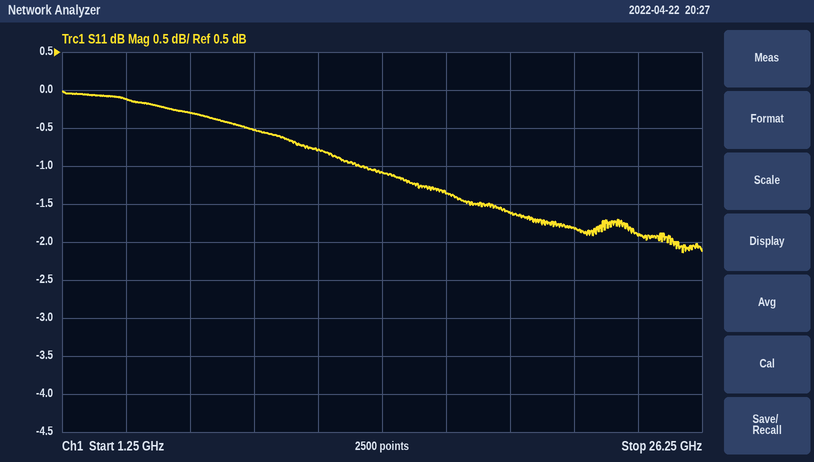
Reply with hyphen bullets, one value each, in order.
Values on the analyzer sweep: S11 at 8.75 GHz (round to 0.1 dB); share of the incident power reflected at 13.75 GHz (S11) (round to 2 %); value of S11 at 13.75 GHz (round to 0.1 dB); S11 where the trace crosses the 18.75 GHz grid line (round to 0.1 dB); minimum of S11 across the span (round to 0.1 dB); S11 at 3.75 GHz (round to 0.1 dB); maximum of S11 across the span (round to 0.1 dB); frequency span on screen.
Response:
- -0.5 dB
- 78 %
- -1.1 dB
- -1.6 dB
- -2.1 dB
- -0.1 dB
- 0.0 dB
- 25 GHz
